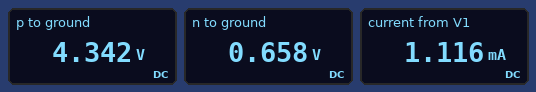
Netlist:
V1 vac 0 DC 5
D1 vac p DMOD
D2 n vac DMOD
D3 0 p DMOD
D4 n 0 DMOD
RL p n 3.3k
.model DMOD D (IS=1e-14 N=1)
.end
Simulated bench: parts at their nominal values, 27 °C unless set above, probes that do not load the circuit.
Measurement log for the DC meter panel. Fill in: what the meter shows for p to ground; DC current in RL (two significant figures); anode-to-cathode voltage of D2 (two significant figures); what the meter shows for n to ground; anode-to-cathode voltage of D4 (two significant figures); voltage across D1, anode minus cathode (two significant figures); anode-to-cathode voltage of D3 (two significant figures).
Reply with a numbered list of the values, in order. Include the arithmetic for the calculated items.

1. 4.342 V
2. (4.342 V - 658 mV) / 3.3 kΩ = 1.1 mA
3. 658 mV - 5 V = -4.3 V
4. 0.658 V
5. 658 mV = 660 mV
6. 5 V - 4.342 V = 660 mV
7. 0 V - 4.342 V = -4.3 V
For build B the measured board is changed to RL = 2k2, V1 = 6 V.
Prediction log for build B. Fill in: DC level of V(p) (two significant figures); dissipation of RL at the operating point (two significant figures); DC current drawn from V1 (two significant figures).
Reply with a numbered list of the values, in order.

1. 5.3 V
2. 9.8 mW
3. 2.1 mA
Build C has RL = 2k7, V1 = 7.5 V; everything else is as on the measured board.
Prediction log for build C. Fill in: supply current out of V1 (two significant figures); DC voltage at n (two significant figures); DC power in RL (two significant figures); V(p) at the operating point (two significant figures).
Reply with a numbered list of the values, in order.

1. 2.3 mA
2. 680 mV
3. 14 mW
4. 6.8 V
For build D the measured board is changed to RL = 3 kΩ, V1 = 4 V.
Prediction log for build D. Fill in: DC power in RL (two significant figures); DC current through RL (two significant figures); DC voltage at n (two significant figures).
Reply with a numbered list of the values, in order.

1. 2.4 mW
2. 900 µA
3. 650 mV
